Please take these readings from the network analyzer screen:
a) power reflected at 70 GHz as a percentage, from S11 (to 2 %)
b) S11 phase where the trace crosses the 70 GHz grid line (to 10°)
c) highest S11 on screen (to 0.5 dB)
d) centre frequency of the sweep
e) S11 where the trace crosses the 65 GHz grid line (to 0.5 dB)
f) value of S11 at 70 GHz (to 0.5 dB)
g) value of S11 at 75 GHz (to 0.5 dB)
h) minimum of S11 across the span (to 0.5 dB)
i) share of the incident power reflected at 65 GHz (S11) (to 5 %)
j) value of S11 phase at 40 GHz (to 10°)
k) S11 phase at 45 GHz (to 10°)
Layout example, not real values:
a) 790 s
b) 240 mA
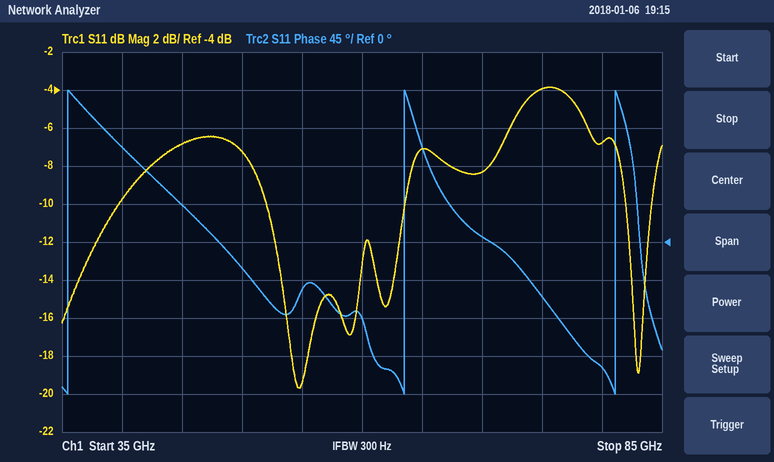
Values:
a) 14 %
b) 10°
c) -4.0 dB
d) 60 GHz
e) -7.0 dB
f) -8.5 dB
g) -4.0 dB
h) -19.5 dB
i) 20 %
j) 110°
k) 40°
